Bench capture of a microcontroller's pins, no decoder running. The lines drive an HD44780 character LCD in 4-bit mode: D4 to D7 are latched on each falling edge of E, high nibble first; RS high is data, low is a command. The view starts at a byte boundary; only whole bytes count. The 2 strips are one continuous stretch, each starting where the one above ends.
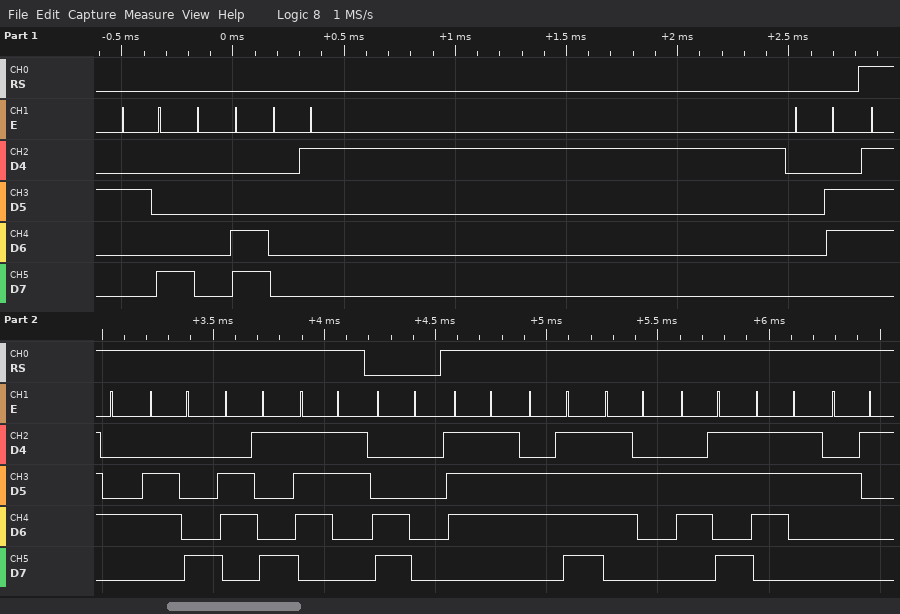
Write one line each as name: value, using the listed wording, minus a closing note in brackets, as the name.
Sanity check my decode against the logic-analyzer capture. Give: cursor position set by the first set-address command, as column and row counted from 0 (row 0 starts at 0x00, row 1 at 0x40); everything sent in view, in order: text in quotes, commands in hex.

cursor position set by the first set-address command, as column and row counted from 0: column 0, row 1
everything sent in view, in order: text in quotes, commands in hex: 0x28 0x0C 0x01 0x06 "this" 0xC0 "works!"
